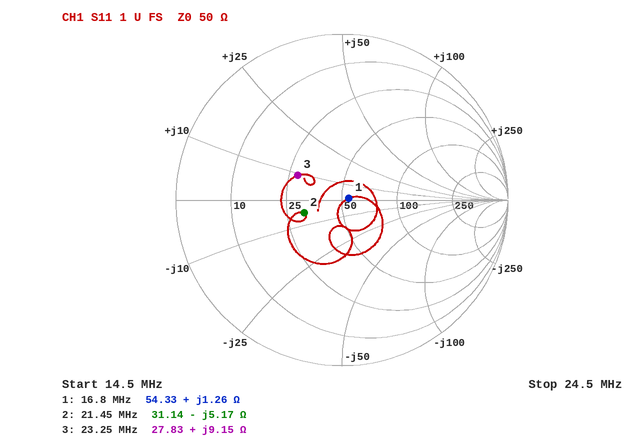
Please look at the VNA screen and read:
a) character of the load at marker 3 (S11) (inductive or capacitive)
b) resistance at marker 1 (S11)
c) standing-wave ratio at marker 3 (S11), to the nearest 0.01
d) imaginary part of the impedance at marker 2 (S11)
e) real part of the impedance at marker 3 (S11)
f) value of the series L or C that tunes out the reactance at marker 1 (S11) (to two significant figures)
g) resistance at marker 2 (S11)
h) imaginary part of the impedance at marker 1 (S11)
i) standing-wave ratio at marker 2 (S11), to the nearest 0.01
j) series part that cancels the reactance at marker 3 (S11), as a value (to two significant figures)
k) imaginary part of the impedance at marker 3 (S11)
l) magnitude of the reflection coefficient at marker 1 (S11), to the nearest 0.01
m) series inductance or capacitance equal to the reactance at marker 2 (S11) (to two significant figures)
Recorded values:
inductive
54.33 Ω
1.88
-5.17 Ω
27.83 Ω
7.5 nF
31.14 Ω
+1.26 Ω
1.63
750 pF
+9.15 Ω
0.04
1.4 nF
